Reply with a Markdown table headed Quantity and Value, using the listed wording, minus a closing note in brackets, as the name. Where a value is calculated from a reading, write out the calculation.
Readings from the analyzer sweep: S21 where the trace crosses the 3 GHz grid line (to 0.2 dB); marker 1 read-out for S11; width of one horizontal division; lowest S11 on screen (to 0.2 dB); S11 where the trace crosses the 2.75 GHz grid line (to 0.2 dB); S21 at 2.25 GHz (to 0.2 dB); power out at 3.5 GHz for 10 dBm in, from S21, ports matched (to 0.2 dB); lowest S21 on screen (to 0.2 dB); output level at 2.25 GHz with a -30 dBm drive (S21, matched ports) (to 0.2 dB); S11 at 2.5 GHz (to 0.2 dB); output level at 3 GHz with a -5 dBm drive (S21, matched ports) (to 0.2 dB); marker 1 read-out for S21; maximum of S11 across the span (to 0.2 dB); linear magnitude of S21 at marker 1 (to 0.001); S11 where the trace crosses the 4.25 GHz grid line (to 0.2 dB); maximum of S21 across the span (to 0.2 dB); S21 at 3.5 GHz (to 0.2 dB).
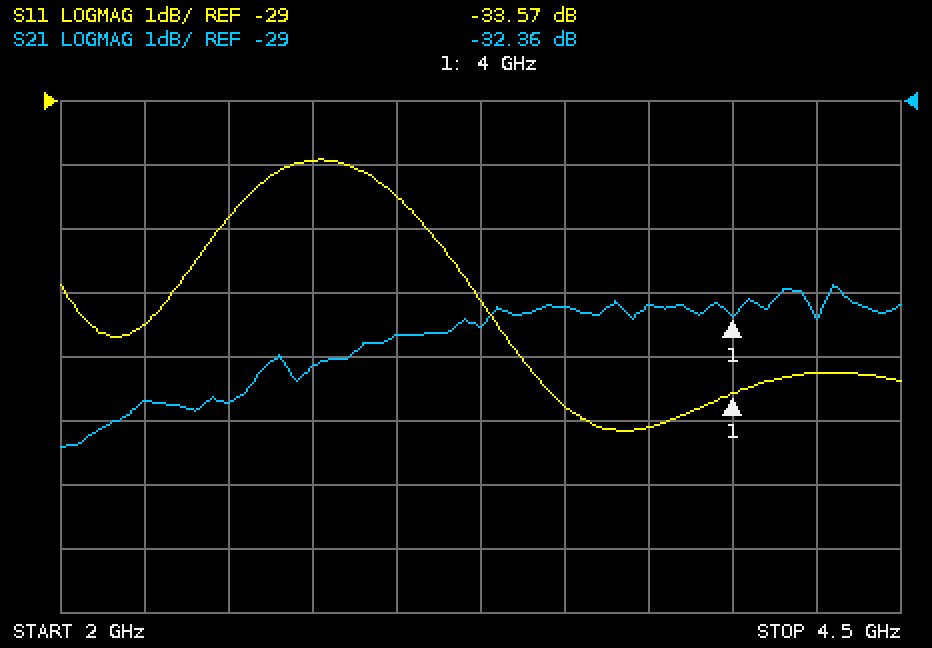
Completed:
| Quantity | Value |
|---|---|
| S21 where the trace crosses the 3 GHz grid line | -32.6 dB |
| marker 1 read-out for S11 | -33.57 dB |
| width of one horizontal division | 250 MHz |
| lowest S11 on screen | -34.2 dB |
| S11 where the trace crosses the 2.75 GHz grid line | -30.0 dB |
| S21 at 2.25 GHz | -33.6 dB |
| power out at 3.5 GHz for 10 dBm in, from S21, ports matched | 10 dBm + (-32.2 dB) = -22.2 dBm |
| lowest S21 on screen | -34.4 dB |
| output level at 2.25 GHz with a -30 dBm drive (S21, matched ports) | -30 dBm + (-33.6 dB) = -63.6 dBm |
| S11 at 2.5 GHz | -30.8 dB |
| output level at 3 GHz with a -5 dBm drive (S21, matched ports) | -5 dBm + (-32.6 dB) = -37.6 dBm |
| marker 1 read-out for S21 | -32.36 dB |
| maximum of S11 across the span | -30.0 dB |
| linear magnitude of S21 at marker 1 | 10^(-32.36/20) ≈ 0.024 |
| S11 where the trace crosses the 4.25 GHz grid line | -33.2 dB |
| maximum of S21 across the span | -31.8 dB |
| S21 at 3.5 GHz | -32.2 dB |
